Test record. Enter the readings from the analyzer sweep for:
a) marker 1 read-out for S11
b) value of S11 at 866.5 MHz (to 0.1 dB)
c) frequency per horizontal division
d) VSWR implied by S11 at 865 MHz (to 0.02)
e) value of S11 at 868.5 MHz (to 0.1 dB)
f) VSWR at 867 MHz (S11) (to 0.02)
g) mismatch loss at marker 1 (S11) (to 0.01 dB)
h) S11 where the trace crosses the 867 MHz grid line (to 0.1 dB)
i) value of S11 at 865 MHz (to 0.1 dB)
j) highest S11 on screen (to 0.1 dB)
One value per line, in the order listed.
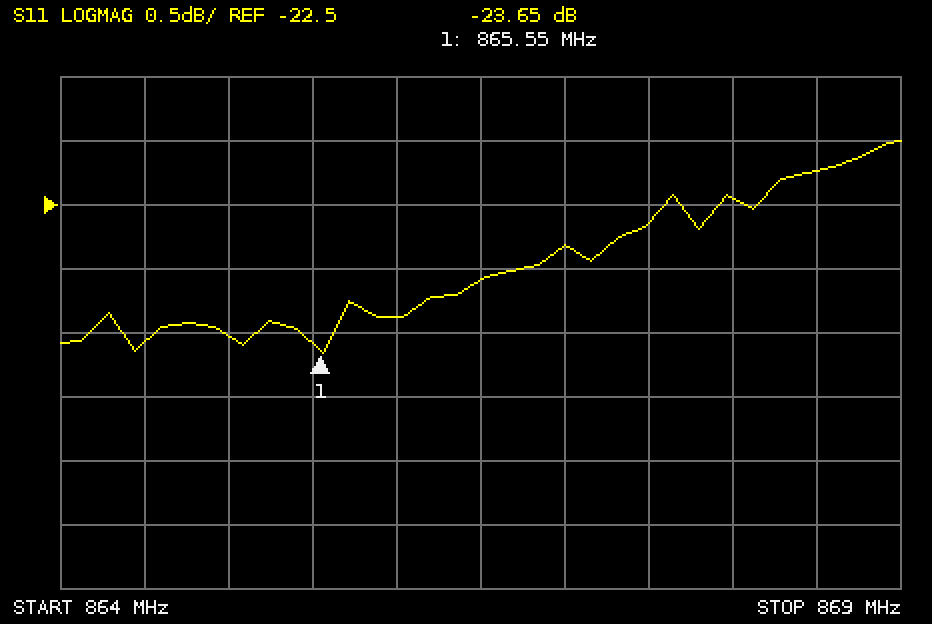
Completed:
-23.65 dB
-23.1 dB
500 kHz
1.14
-22.2 dB
1.16
0.02 dB
-22.8 dB
-23.5 dB
-22.0 dB
